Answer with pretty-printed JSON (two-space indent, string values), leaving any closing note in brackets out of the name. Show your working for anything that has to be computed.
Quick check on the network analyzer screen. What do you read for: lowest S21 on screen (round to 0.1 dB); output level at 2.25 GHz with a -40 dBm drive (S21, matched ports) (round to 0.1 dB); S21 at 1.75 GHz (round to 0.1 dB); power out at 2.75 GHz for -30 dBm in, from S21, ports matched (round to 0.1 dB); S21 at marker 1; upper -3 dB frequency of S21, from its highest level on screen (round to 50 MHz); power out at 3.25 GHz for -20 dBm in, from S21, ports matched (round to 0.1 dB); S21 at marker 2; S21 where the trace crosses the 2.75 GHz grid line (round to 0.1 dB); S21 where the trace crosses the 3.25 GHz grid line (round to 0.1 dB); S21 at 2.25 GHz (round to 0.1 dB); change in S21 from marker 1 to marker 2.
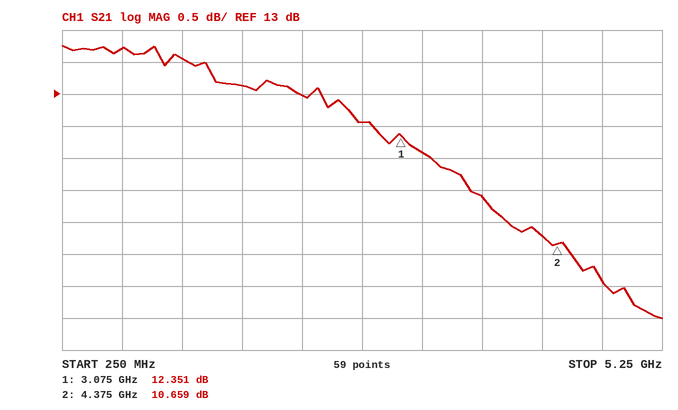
{
  "lowest S21 on screen": "9.5 dB",
  "output level at 2.25 GHz with a -40 dBm drive (S21, matched ports)": "-40 dBm + (13.0 dB) = -27.0 dBm",
  "S21 at 1.75 GHz": "13.1 dB",
  "power out at 2.75 GHz for -30 dBm in, from S21, ports matched": "-30 dBm + (12.6 dB) = -17.4 dBm",
  "S21 at marker 1": "12.351 dB",
  "upper -3 dB frequency of S21, from its highest level on screen": "4.25 GHz",
  "power out at 3.25 GHz for -20 dBm in, from S21, ports matched": "-20 dBm + (12.1 dB) = -7.9 dBm",
  "S21 at marker 2": "10.659 dB",
  "S21 where the trace crosses the 2.75 GHz grid line": "12.6 dB",
  "S21 where the trace crosses the 3.25 GHz grid line": "12.1 dB",
  "S21 at 2.25 GHz": "13.0 dB",
  "change in S21 from marker 1 to marker 2": "10.659 − (12.351) = -1.692 dB"
}
